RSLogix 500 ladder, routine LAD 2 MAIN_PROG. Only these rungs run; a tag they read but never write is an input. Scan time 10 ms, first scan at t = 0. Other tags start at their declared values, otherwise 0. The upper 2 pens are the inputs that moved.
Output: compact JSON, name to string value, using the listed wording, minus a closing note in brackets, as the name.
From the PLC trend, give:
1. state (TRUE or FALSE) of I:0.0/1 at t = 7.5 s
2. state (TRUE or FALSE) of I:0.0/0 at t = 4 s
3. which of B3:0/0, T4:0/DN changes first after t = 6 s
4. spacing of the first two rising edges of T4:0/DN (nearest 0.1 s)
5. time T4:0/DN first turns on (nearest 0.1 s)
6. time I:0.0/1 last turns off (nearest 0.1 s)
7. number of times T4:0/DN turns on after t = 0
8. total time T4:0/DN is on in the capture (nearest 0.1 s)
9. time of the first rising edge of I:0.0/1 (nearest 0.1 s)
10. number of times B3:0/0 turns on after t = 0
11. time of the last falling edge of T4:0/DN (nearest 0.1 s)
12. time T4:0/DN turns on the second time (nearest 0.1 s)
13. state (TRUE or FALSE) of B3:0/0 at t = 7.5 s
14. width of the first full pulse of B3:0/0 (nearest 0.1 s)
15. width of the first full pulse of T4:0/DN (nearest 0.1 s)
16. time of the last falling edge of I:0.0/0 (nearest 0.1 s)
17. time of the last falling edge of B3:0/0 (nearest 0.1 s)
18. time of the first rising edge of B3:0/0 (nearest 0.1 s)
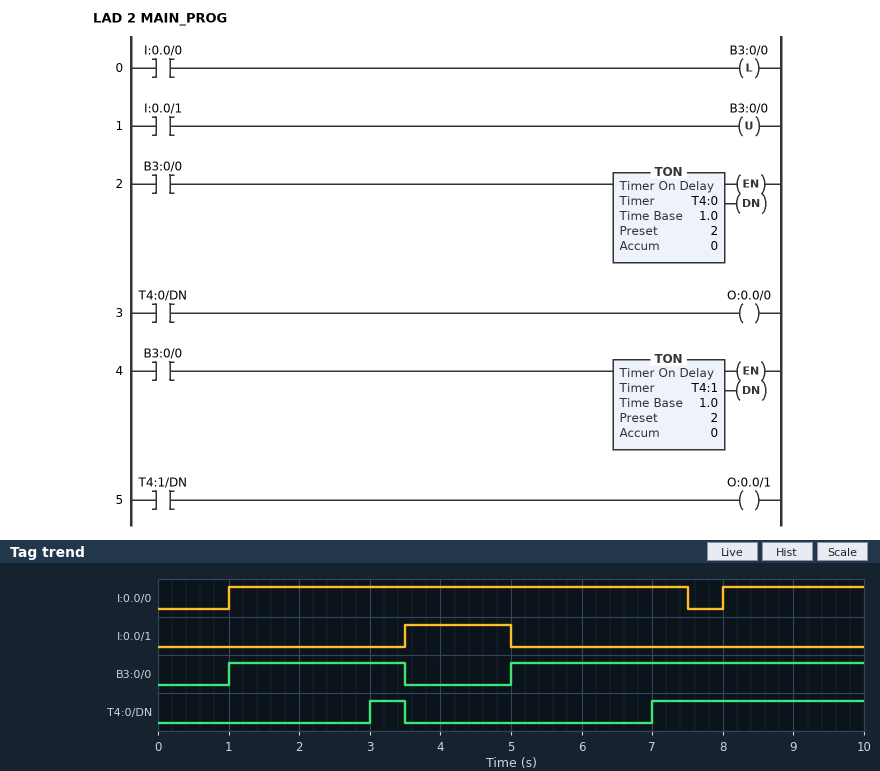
{"state (TRUE or FALSE) of I:0.0/1 at t = 7.5 s": "FALSE", "state (TRUE or FALSE) of I:0.0/0 at t = 4 s": "TRUE", "which of B3:0/0, T4:0/DN changes first after t = 6 s": "T4:0/DN", "spacing of the first two rising edges of T4:0/DN": "4.0 s", "time T4:0/DN first turns on": "3.0 s", "time I:0.0/1 last turns off": "5.0 s", "number of times T4:0/DN turns on after t = 0": "2", "total time T4:0/DN is on in the capture": "3.5 s", "time of the first rising edge of I:0.0/1": "3.5 s", "number of times B3:0/0 turns on after t = 0": "2", "time of the last falling edge of T4:0/DN": "3.5 s", "time T4:0/DN turns on the second time": "7.0 s", "state (TRUE or FALSE) of B3:0/0 at t = 7.5 s": "TRUE", "width of the first full pulse of B3:0/0": "2.5 s", "width of the first full pulse of T4:0/DN": "0.5 s", "time of the last falling edge of I:0.0/0": "7.5 s", "time of the last falling edge of B3:0/0": "3.5 s", "time of the first rising edge of B3:0/0": "1.0 s"}
